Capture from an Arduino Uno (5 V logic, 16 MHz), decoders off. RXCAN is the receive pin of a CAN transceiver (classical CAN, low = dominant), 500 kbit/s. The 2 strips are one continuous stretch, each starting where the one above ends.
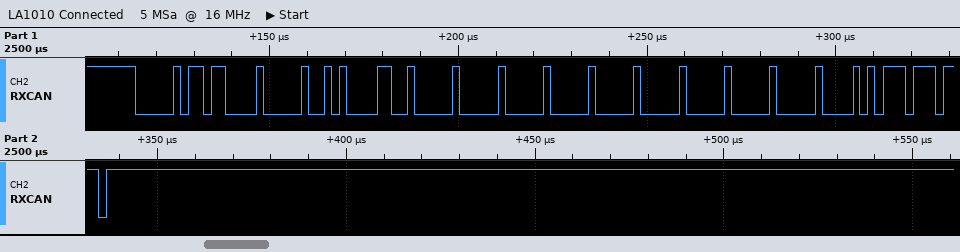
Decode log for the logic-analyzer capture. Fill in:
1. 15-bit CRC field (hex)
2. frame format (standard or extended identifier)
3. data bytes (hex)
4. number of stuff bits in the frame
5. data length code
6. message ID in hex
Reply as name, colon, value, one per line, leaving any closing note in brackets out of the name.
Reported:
15-bit CRC field: 0x2BBB
frame format: standard
data bytes: 0A 19 00 00 00 00 00 00
number of stuff bits in the frame: 11
data length code: 8
message ID in hex: 0x036
